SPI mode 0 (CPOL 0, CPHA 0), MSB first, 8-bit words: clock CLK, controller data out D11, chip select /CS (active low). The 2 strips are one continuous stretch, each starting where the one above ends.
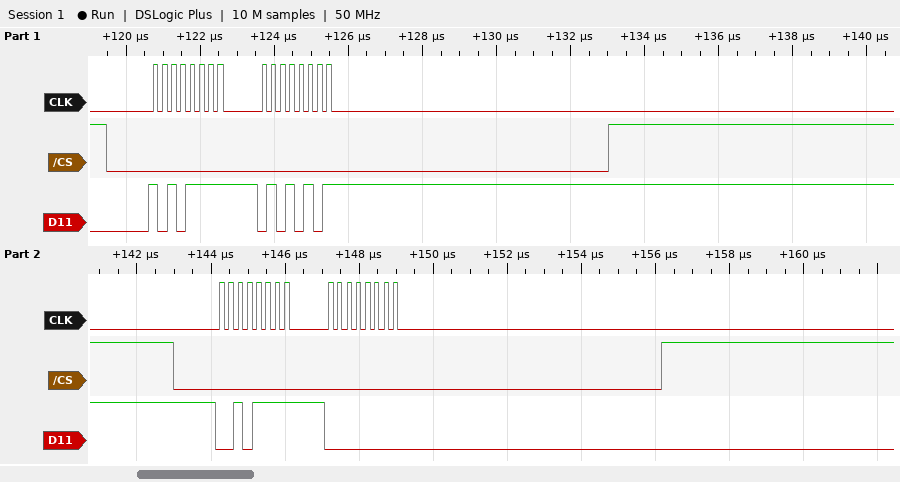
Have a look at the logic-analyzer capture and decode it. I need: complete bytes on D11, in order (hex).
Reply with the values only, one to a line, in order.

AF 55 2F 00
